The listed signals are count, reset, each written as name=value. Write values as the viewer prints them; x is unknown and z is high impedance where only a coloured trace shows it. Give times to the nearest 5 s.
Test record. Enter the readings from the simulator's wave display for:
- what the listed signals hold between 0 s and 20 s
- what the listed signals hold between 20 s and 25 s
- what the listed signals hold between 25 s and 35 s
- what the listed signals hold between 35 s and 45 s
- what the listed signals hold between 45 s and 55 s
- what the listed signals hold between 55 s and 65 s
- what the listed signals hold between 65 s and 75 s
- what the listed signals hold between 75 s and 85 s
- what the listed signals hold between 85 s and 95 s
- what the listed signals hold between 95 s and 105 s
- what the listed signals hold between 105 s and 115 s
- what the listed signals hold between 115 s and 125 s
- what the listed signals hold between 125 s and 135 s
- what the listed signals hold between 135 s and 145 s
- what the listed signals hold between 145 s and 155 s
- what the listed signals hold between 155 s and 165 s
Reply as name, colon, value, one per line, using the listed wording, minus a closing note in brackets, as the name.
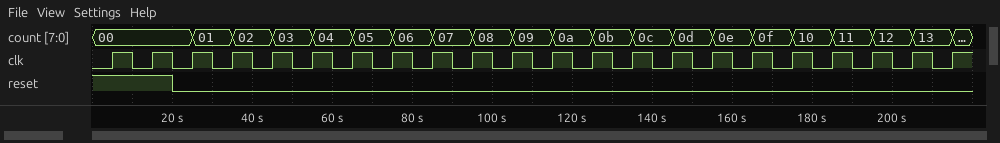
what the listed signals hold between 0 s and 20 s: count=00, reset=1
what the listed signals hold between 20 s and 25 s: count=00, reset=0
what the listed signals hold between 25 s and 35 s: count=01, reset=0
what the listed signals hold between 35 s and 45 s: count=02, reset=0
what the listed signals hold between 45 s and 55 s: count=03, reset=0
what the listed signals hold between 55 s and 65 s: count=04, reset=0
what the listed signals hold between 65 s and 75 s: count=05, reset=0
what the listed signals hold between 75 s and 85 s: count=06, reset=0
what the listed signals hold between 85 s and 95 s: count=07, reset=0
what the listed signals hold between 95 s and 105 s: count=08, reset=0
what the listed signals hold between 105 s and 115 s: count=09, reset=0
what the listed signals hold between 115 s and 125 s: count=0a, reset=0
what the listed signals hold between 125 s and 135 s: count=0b, reset=0
what the listed signals hold between 135 s and 145 s: count=0c, reset=0
what the listed signals hold between 145 s and 155 s: count=0d, reset=0
what the listed signals hold between 155 s and 165 s: count=0e, reset=0
